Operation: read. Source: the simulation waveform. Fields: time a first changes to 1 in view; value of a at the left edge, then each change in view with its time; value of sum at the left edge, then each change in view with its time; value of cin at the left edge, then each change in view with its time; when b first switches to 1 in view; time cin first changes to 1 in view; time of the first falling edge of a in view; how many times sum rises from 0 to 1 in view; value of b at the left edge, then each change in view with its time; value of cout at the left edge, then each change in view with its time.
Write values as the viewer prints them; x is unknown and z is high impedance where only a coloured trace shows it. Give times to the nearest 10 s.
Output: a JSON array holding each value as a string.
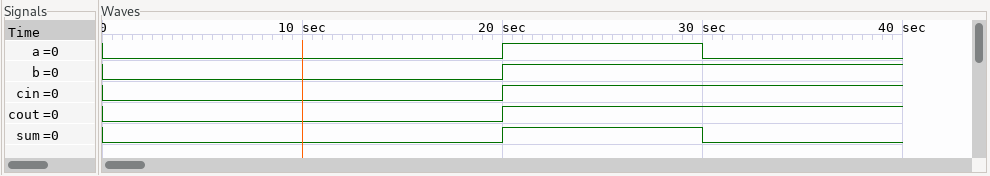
["20 s", "0, 1 at 20 s, 0 at 30 s", "0, 1 at 20 s, 0 at 30 s", "0, 1 at 20 s", "20 s", "20 s", "30 s", "1", "0, 1 at 20 s", "0, 1 at 20 s"]
